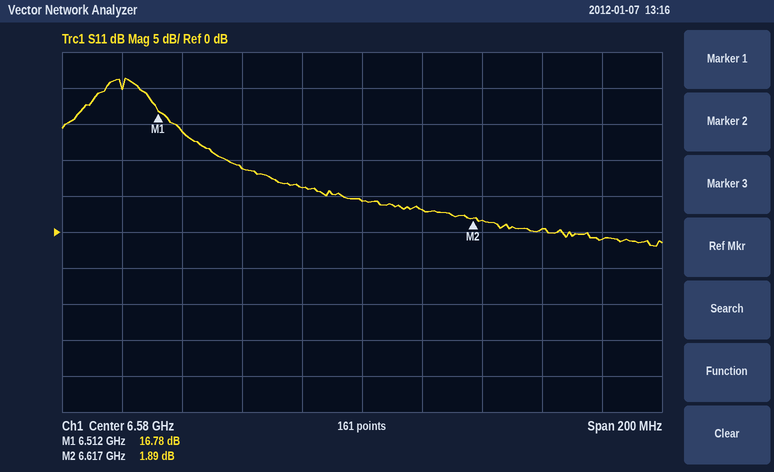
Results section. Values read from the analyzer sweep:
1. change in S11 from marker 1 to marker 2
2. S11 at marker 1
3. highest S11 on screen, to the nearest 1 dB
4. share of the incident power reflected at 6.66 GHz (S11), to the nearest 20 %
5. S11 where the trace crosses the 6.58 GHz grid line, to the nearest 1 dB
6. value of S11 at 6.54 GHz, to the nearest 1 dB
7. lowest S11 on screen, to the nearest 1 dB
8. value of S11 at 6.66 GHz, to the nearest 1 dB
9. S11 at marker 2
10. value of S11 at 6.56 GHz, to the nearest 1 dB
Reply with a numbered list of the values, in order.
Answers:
1. -14.89 dB
2. 16.78 dB
3. 21 dB
4. 80 %
5. 4 dB
6. 9 dB
7. -2 dB
8. -1 dB
9. 1.89 dB
10. 6 dB
